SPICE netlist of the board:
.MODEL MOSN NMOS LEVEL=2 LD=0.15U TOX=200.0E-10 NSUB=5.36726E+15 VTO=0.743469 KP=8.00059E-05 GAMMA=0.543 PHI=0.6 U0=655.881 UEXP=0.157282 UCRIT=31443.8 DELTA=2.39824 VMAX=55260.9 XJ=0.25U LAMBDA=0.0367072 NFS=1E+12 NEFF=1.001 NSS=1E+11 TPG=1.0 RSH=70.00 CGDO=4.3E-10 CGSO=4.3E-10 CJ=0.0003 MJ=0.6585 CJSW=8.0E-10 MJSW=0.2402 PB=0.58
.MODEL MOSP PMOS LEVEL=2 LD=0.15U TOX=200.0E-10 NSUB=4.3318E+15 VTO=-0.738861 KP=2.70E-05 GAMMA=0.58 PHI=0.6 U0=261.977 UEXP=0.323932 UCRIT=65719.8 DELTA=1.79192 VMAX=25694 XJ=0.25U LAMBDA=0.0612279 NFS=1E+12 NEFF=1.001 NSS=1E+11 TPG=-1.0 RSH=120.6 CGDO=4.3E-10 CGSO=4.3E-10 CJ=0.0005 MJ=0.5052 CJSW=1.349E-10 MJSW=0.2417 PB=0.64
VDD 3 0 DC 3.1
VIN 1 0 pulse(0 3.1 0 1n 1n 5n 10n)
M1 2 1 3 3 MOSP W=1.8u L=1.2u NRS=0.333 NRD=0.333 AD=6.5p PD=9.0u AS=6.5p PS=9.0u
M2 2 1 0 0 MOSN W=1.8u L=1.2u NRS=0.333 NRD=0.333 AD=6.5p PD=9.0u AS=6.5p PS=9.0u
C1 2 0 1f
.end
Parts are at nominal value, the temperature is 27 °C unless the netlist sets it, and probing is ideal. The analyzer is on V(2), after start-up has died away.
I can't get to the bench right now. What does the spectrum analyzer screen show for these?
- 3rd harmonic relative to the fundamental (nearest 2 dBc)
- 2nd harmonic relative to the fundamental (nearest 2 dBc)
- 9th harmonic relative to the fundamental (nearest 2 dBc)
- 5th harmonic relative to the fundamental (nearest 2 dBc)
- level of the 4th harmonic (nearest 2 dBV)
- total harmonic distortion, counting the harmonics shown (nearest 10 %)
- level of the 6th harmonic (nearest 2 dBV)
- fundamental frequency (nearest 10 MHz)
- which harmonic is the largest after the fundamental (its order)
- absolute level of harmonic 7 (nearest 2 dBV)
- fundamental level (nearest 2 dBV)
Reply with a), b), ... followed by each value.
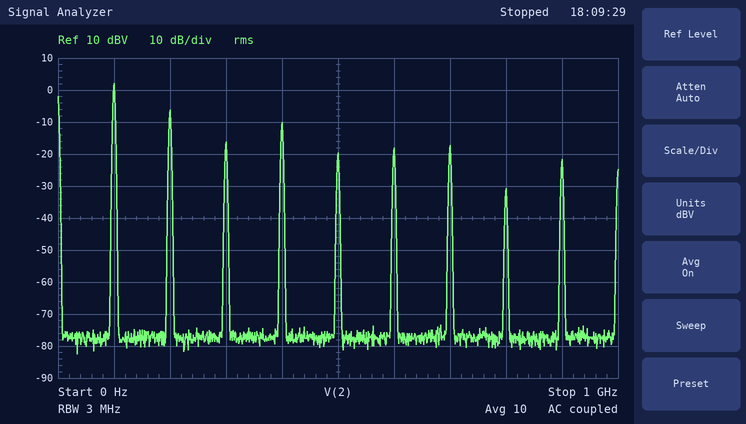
a) -18 dBc
b) -8 dBc
c) -24 dBc
d) -22 dBc
e) -10 dBV
f) 50 %
g) -18 dBV
h) 100 MHz
i) 2
j) -18 dBV
k) 2 dBV
